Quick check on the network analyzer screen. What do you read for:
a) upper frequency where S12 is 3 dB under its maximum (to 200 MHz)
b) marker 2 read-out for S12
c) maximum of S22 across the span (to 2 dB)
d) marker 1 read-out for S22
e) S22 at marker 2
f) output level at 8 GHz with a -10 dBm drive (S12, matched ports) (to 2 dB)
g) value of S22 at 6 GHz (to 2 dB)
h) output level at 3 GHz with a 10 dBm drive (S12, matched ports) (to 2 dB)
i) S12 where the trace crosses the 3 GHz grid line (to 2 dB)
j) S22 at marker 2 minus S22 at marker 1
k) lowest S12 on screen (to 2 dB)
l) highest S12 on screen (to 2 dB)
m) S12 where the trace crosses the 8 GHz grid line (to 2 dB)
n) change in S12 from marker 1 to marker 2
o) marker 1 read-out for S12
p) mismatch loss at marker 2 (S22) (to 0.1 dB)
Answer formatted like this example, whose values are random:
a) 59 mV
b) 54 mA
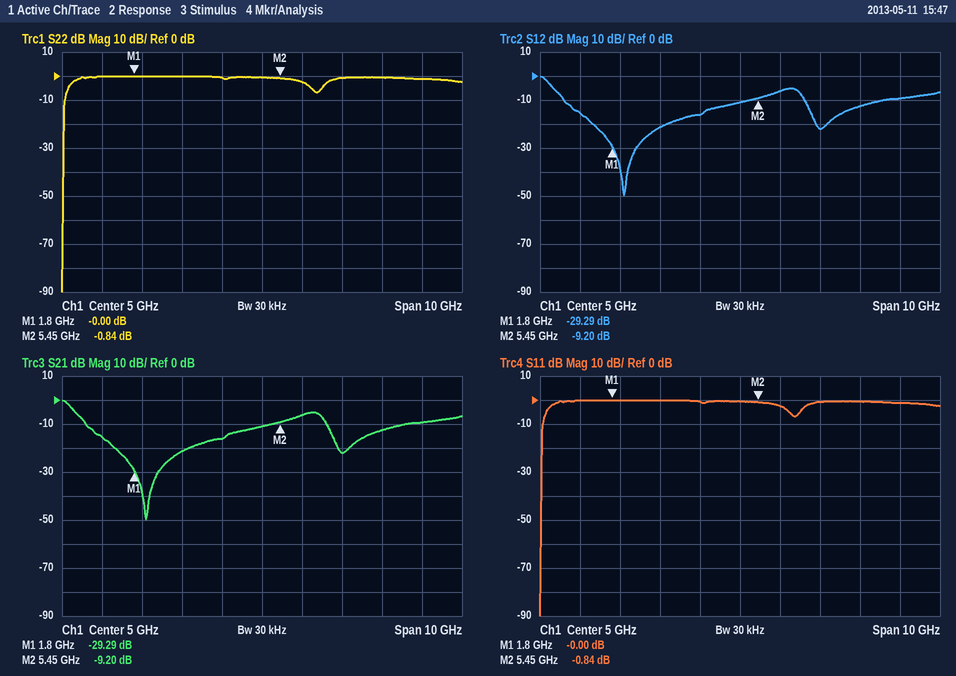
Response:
a) 200 MHz
b) -9.20 dB
c) 0 dB
d) -0.00 dB
e) -0.84 dB
f) -22 dBm
g) -2 dB
h) -12 dBm
i) -22 dB
j) -0.84 dB
k) -50 dB
l) 0 dB
m) -12 dB
n) 20.09 dB
o) -29.29 dB
p) 7.5 dB
